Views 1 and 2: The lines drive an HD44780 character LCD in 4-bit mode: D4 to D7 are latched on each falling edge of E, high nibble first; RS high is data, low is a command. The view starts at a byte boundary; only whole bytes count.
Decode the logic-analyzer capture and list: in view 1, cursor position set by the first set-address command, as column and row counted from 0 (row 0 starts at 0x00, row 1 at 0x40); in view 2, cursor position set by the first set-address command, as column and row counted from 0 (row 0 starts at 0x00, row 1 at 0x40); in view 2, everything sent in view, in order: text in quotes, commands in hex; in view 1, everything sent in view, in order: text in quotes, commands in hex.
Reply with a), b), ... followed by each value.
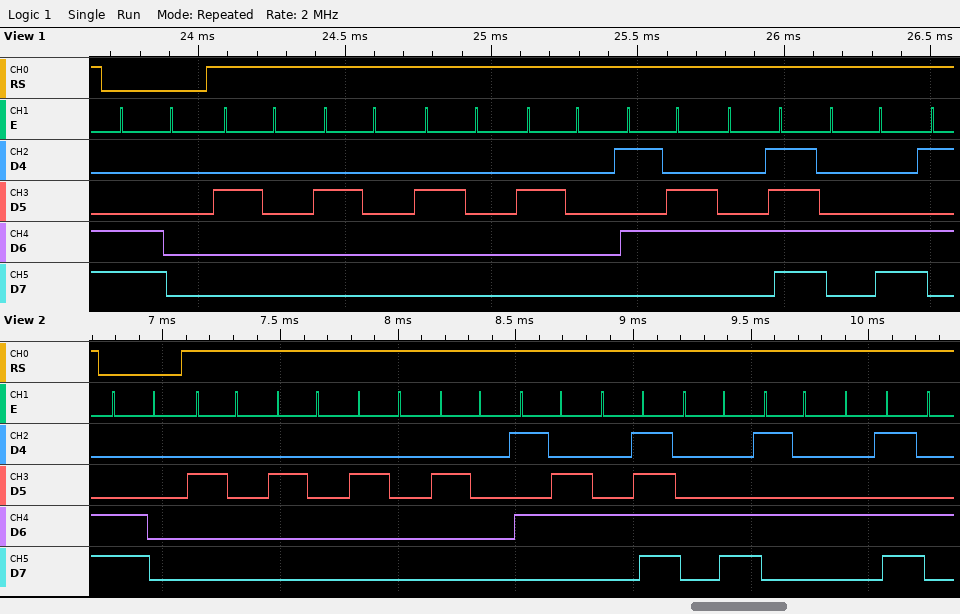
a) column 0, row 1
b) column 0, row 1
c) 0xC0 "    VOLTM"
d) 0xC0 "    VOL"
